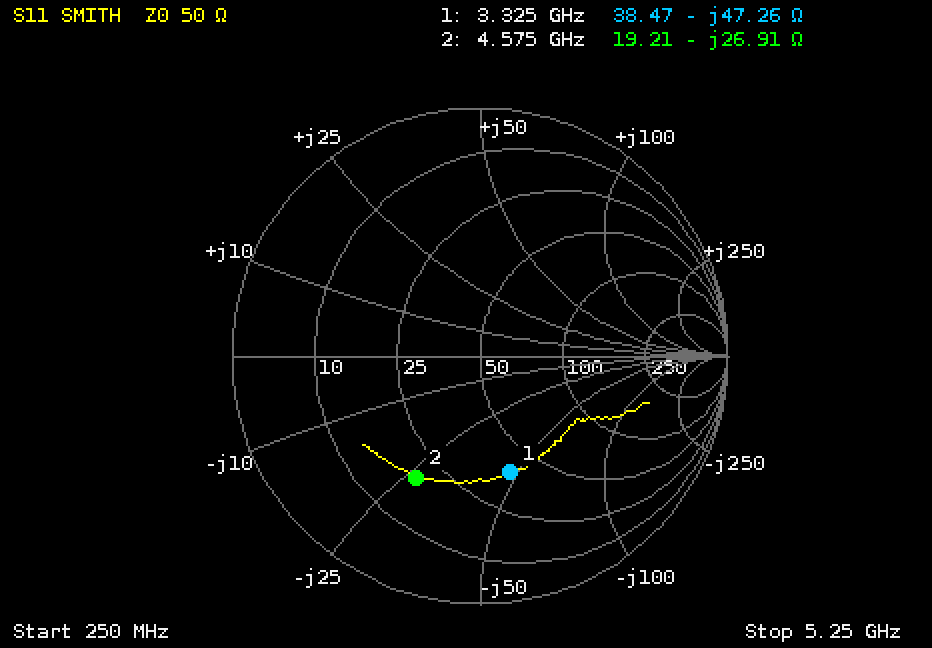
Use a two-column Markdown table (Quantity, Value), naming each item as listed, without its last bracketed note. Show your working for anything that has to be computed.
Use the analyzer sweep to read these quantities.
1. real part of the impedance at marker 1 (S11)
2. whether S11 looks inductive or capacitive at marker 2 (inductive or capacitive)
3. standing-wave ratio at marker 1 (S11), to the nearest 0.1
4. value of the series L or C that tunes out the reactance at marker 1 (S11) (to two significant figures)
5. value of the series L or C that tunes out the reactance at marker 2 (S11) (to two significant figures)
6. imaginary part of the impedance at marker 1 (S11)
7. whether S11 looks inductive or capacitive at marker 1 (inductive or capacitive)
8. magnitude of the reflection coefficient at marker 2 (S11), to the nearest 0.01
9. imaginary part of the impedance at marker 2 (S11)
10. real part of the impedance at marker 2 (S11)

| Quantity | Value |
|---|---|
| real part of the impedance at marker 1 | 38.47 Ω |
| whether S11 looks inductive or capacitive at marker 2 | capacitive |
| standing-wave ratio at marker 1 (S11), to the nearest 0.1 | 2.9 |
| value of the series L or C that tunes out the reactance at marker 1 (S11) | L = 47.26 Ω/(2π × 3.325 GHz) ≈ 2.3 nH |
| value of the series L or C that tunes out the reactance at marker 2 (S11) | L = 26.91 Ω/(2π × 4.575 GHz) ≈ 936 pH, so 940 pH to two significant figures |
| imaginary part of the impedance at marker 1 | -47.26 Ω |
| whether S11 looks inductive or capacitive at marker 1 | capacitive |
| magnitude of the reflection coefficient at marker 2 (S11), to the nearest 0.01 | 0.55 |
| imaginary part of the impedance at marker 2 | -26.91 Ω |
| real part of the impedance at marker 2 | 19.21 Ω |
